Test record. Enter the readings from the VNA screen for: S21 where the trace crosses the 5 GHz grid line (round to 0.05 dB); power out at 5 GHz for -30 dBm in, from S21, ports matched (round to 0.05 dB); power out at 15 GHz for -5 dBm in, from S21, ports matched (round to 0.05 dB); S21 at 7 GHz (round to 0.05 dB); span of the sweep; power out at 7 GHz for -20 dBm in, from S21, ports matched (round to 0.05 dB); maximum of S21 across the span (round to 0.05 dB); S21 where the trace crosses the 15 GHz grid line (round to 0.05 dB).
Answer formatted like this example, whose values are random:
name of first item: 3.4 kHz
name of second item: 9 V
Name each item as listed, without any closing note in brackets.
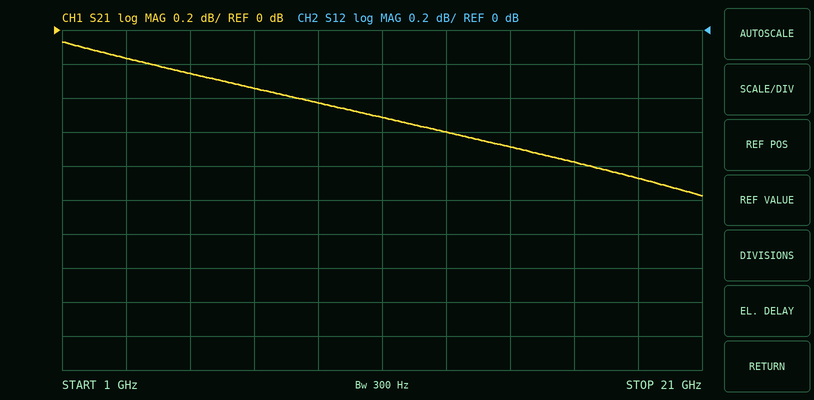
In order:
S21 where the trace crosses the 5 GHz grid line: -0.25 dB
power out at 5 GHz for -30 dBm in, from S21, ports matched: -30.25 dBm
power out at 15 GHz for -5 dBm in, from S21, ports matched: -5.70 dBm
S21 at 7 GHz: -0.35 dB
span of the sweep: 20 GHz
power out at 7 GHz for -20 dBm in, from S21, ports matched: -20.35 dBm
maximum of S21 across the span: -0.05 dB
S21 where the trace crosses the 15 GHz grid line: -0.70 dB
